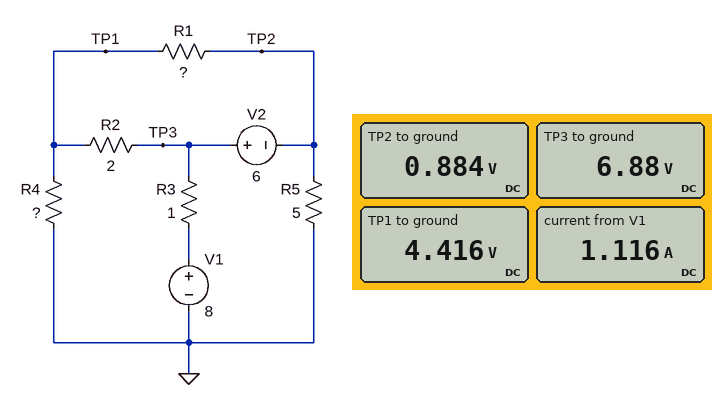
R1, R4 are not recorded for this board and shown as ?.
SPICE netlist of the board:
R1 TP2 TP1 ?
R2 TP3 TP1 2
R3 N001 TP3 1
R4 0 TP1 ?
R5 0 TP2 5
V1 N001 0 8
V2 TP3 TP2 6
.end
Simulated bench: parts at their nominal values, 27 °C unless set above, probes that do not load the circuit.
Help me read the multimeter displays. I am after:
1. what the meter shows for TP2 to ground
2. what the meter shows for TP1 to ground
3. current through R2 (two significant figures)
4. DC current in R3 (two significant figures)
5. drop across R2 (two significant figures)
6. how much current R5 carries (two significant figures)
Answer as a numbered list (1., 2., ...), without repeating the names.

1. 0.884 V
2. 4.416 V
3. 1.2 A
4. 1.1 A
5. 2.5 V
6. 180 mA
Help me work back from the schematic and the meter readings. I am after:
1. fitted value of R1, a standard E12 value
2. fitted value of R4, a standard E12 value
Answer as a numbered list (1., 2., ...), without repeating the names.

1. 12 Ω
2. 4.7 Ω
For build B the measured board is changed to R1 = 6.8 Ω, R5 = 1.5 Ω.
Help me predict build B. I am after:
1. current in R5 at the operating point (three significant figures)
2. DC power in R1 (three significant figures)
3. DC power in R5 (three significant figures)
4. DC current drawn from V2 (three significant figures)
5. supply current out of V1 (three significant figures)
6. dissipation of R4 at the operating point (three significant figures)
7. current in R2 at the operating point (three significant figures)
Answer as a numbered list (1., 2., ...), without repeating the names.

1. 459 mA
2. 1.62 W
3. 316 mW
4. 29.1 mA
5. 1.31 A
6. 3.42 W
7. 1.34 A
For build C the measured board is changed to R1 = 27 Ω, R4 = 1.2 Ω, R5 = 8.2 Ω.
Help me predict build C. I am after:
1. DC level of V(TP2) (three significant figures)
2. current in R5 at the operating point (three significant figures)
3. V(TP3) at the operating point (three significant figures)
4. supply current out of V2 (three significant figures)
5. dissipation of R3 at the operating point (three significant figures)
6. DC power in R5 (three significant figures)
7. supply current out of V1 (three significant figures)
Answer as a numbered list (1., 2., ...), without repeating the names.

1. 121 mV
2. 14.8 mA
3. 6.12 V
4. 63.6 mA
5. 3.53 W
6. 1.79 mW
7. 1.88 A
